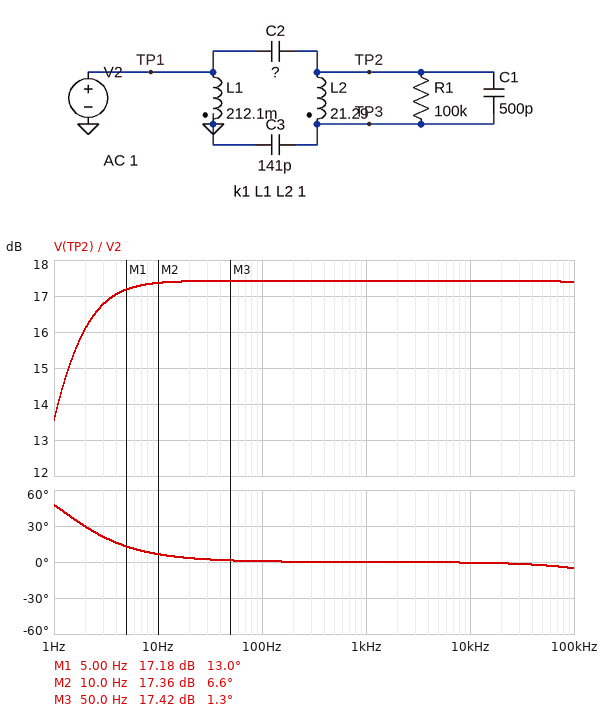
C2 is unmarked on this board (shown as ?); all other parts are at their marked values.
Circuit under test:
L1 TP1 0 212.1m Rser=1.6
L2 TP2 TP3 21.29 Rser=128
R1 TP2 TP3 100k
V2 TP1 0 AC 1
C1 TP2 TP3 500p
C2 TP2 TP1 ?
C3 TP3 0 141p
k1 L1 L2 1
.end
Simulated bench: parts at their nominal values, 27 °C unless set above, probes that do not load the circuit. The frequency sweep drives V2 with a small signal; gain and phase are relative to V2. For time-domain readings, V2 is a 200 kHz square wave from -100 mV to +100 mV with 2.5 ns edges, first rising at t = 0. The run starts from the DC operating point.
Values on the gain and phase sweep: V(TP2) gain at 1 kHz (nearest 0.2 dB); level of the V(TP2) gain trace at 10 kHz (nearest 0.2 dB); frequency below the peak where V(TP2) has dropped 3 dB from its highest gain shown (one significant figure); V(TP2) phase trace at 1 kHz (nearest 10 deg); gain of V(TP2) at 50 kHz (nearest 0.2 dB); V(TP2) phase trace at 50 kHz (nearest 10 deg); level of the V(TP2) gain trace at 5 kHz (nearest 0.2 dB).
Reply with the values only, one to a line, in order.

17.4 dB
17.4 dB
1 Hz
0 deg
17.4 dB
0 deg
17.4 dB
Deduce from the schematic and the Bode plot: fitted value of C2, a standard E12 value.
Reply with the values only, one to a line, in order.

56 pF
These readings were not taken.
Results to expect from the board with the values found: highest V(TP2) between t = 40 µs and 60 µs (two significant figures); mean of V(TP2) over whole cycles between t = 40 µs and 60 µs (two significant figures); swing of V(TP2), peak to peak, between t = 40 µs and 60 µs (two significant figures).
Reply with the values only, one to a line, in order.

1.5 V
740 mV
1.5 V
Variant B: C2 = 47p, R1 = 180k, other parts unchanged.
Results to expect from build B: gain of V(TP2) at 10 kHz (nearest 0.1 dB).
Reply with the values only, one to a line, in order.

17.8 dB
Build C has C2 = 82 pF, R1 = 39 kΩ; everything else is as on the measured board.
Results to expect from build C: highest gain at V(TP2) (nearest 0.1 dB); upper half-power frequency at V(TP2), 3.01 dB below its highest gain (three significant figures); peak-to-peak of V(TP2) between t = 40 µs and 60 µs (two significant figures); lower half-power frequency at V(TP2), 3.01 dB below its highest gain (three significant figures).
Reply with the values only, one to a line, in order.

16.5 dB
1.01 MHz
1.3 V
1.19 Hz
